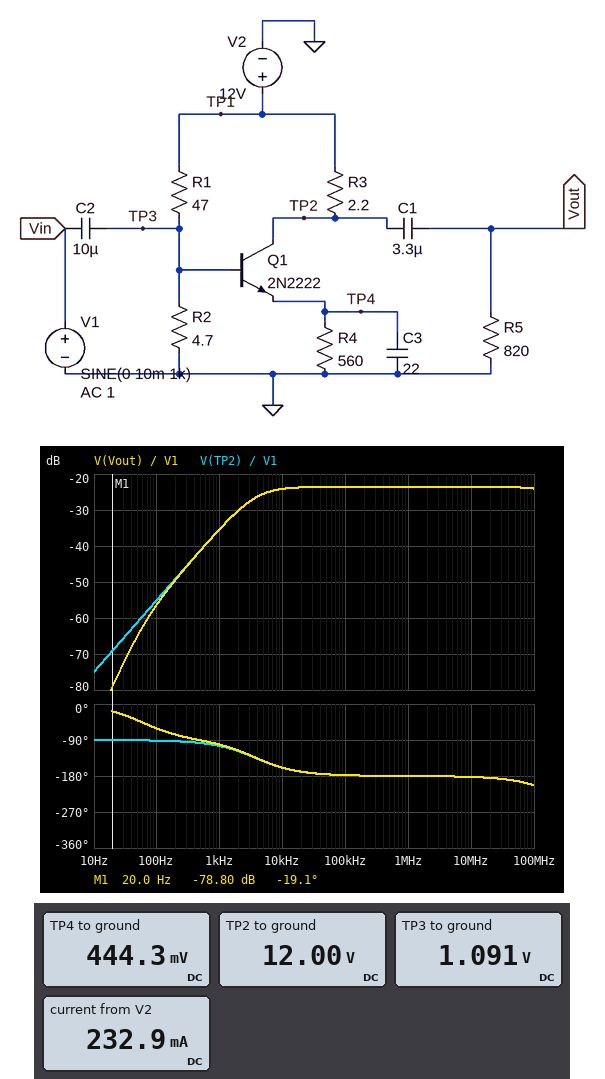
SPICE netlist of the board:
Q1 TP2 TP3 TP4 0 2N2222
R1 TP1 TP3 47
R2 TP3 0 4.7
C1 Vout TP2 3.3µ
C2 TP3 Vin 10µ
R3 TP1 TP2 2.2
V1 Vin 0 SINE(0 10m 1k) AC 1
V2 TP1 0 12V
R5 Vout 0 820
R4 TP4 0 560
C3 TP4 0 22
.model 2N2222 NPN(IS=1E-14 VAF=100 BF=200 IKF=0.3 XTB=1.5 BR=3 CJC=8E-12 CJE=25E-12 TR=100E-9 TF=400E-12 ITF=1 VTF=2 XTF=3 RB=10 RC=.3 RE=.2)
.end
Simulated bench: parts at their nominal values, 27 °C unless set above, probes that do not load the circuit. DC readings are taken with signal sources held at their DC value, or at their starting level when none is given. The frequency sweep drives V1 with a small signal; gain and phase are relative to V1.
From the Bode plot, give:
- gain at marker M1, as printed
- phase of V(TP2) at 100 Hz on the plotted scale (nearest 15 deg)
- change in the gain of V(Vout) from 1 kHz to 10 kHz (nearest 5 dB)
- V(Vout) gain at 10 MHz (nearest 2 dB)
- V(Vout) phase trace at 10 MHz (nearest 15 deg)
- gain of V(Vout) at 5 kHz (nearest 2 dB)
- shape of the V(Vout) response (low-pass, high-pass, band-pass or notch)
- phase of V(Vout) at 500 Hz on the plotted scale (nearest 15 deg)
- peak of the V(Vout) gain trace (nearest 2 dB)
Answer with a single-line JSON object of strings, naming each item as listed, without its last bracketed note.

{"gain at marker M1, as printed": "-78.80 dB", "phase of V(TP2) at 100 Hz on the plotted scale": "-90 deg", "change in the gain of V(Vout) from 1 kHz to 10 kHz": "10 dB", "V(Vout) gain at 10 MHz": "-24 dB", "V(Vout) phase trace at 10 MHz": "-180 deg", "gain of V(Vout) at 5 kHz": "-26 dB", "shape of the V(Vout) response": "high-pass", "phase of V(Vout) at 500 Hz on the plotted scale": "-90 deg", "peak of the V(Vout) gain trace": "-24 dB"}
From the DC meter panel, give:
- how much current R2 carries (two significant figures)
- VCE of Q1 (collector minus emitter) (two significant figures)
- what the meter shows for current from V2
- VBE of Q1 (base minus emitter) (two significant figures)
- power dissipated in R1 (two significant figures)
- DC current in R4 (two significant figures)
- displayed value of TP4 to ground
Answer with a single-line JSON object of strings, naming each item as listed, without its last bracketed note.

{"how much current R2 carries": "230 mA", "VCE of Q1 (collector minus emitter)": "12 V", "what the meter shows for current from V2": "232.9 mA", "VBE of Q1 (base minus emitter)": "650 mV", "power dissipated in R1": "2.5 W", "DC current in R4": "790 µA", "displayed value of TP4 to ground": "444.3 mV"}
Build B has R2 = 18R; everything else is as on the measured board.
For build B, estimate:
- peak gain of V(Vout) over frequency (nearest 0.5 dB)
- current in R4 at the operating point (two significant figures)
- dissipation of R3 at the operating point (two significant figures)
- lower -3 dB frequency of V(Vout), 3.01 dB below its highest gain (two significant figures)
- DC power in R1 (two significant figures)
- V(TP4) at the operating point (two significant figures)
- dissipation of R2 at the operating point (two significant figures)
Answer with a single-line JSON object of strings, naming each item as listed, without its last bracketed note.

{"peak gain of V(Vout) over frequency": "-8.5 dB", "current in R4 at the operating point": "4.7 mA", "dissipation of R3 at the operating point": "48 µW", "lower -3 dB frequency of V(Vout), 3.01 dB below its highest gain": "1.2 kHz", "DC power in R1": "1.6 W", "V(TP4) at the operating point": "2.6 V", "dissipation of R2 at the operating point": "610 mW"}
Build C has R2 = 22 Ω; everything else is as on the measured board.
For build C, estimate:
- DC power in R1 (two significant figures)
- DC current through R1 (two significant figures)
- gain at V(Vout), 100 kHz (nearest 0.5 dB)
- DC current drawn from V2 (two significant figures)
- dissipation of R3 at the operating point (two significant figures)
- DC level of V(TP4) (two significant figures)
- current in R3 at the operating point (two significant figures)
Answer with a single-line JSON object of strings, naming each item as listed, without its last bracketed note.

{"DC power in R1": "1.4 W", "DC current through R1": "170 mA", "gain at V(Vout), 100 kHz": "-7.0 dB", "DC current drawn from V2": "180 mA", "dissipation of R3 at the operating point": "68 µW", "DC level of V(TP4)": "3.1 V", "current in R3 at the operating point": "5.6 mA"}
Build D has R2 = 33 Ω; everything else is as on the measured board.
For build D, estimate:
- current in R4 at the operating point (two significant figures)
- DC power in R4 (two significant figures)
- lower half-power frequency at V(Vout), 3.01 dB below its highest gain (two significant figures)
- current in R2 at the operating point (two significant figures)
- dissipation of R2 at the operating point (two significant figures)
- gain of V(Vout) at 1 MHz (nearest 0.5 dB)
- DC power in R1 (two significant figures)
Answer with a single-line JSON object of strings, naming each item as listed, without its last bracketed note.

{"current in R4 at the operating point": "7.6 mA", "DC power in R4": "32 mW", "lower half-power frequency at V(Vout), 3.01 dB below its highest gain": "850 Hz", "current in R2 at the operating point": "150 mA", "dissipation of R2 at the operating point": "740 mW", "gain of V(Vout) at 1 MHz": "-4.5 dB", "DC power in R1": "1.1 W"}
